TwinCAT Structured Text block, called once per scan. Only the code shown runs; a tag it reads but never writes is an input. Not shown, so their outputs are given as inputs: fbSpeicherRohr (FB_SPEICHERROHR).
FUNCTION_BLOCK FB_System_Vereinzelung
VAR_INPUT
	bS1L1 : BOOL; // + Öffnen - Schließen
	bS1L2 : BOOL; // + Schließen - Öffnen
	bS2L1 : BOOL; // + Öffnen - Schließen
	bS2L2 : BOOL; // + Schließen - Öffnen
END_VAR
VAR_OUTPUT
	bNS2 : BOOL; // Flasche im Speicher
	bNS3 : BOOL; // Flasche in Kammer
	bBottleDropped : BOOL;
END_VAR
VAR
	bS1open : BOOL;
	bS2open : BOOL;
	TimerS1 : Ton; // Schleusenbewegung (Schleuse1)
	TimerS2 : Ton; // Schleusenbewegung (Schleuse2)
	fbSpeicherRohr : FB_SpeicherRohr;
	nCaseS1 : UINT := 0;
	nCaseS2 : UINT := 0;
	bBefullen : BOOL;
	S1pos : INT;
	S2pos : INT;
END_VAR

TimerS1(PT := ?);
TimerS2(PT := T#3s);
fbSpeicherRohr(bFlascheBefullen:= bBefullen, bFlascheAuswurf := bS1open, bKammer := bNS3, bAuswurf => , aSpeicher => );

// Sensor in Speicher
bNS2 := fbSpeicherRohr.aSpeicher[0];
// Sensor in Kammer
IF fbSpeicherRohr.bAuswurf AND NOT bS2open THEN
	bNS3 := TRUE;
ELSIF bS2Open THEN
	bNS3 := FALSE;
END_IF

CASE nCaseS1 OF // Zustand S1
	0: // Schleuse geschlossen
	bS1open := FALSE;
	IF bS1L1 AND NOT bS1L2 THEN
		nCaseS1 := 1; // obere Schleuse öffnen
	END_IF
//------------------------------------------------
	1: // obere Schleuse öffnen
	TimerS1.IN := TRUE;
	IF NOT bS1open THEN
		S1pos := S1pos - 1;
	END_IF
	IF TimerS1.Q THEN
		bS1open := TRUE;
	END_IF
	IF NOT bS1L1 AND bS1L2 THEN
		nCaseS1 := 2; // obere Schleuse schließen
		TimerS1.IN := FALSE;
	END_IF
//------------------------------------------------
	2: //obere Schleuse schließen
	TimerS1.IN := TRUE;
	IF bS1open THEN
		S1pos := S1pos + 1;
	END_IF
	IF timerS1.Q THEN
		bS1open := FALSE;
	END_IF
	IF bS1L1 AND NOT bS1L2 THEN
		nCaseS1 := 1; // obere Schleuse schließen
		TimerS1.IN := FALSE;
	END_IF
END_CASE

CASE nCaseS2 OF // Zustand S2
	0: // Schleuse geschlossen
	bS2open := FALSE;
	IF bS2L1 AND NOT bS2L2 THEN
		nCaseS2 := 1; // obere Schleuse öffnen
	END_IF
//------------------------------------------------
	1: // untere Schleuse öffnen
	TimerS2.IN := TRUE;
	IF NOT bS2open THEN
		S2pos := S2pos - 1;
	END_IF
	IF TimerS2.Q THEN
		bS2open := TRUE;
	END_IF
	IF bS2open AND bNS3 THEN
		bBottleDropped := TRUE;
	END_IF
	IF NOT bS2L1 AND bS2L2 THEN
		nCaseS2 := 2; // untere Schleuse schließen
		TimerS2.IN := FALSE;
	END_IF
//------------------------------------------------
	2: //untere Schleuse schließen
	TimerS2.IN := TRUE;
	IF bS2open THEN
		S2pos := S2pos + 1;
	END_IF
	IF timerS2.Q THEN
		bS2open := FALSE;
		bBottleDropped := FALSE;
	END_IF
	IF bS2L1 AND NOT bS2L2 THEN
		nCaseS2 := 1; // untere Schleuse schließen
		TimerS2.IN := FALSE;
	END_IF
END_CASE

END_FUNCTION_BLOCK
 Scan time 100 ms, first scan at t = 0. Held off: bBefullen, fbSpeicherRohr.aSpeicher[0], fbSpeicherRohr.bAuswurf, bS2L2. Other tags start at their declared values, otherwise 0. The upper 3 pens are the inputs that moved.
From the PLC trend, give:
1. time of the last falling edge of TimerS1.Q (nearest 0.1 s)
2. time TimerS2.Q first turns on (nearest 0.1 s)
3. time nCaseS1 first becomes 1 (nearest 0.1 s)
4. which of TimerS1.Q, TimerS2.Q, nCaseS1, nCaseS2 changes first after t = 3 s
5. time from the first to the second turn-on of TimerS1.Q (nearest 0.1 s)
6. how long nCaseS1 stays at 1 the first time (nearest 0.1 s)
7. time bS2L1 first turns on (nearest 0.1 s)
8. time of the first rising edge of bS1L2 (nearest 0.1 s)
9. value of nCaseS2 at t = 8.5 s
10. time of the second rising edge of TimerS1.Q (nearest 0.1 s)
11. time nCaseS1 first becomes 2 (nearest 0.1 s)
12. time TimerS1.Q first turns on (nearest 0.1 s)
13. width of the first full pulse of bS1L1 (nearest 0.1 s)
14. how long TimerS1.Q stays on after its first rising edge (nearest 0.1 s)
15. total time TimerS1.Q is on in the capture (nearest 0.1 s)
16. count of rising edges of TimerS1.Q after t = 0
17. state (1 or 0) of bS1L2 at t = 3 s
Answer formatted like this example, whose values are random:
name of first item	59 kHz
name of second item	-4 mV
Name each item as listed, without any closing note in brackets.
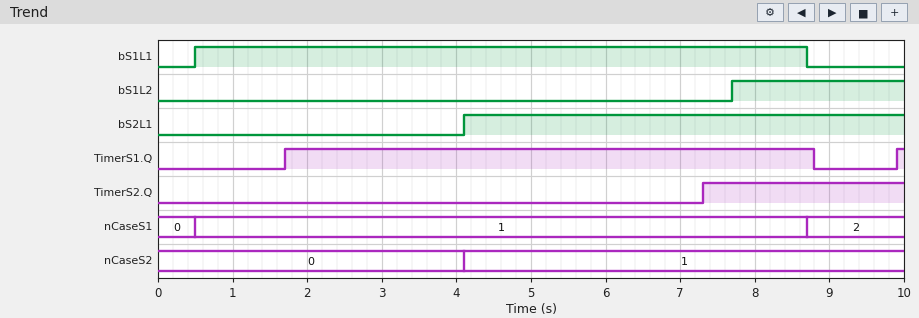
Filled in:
time of the last falling edge of TimerS1.Q	8.8 s
time TimerS2.Q first turns on	7.3 s
time nCaseS1 first becomes 1	0.5 s
which of TimerS1.Q, TimerS2.Q, nCaseS1, nCaseS2 changes first after t = 3 s	nCaseS2
time from the first to the second turn-on of TimerS1.Q	8.2 s
how long nCaseS1 stays at 1 the first time	8.2 s
time bS2L1 first turns on	4.1 s
time of the first rising edge of bS1L2	7.7 s
value of nCaseS2 at t = 8.5 s	1
time of the second rising edge of TimerS1.Q	9.9 s
time nCaseS1 first becomes 2	8.7 s
time TimerS1.Q first turns on	1.7 s
width of the first full pulse of bS1L1	8.2 s
how long TimerS1.Q stays on after its first rising edge	7.1 s
total time TimerS1.Q is on in the capture	7.2 s
count of rising edges of TimerS1.Q after t = 0	2
state (1 or 0) of bS1L2 at t = 3 s	0
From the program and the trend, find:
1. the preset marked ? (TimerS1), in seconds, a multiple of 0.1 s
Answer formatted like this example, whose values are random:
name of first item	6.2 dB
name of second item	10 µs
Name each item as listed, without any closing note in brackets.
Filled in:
the preset marked ? (TimerS1), in seconds, a multiple of 0.1 s	1.0 s
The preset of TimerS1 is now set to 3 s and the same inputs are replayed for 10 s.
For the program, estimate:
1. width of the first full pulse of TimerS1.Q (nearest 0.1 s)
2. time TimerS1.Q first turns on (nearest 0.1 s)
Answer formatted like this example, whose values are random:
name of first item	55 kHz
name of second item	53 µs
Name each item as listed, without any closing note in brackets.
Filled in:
width of the first full pulse of TimerS1.Q	5.1 s
time TimerS1.Q first turns on	3.7 s
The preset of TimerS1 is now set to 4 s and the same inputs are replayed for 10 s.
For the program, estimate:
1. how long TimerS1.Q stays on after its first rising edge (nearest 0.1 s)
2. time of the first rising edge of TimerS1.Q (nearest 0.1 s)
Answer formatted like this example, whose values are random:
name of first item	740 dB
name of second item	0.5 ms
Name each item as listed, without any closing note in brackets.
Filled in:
how long TimerS1.Q stays on after its first rising edge	4.1 s
time of the first rising edge of TimerS1.Q	4.7 s
